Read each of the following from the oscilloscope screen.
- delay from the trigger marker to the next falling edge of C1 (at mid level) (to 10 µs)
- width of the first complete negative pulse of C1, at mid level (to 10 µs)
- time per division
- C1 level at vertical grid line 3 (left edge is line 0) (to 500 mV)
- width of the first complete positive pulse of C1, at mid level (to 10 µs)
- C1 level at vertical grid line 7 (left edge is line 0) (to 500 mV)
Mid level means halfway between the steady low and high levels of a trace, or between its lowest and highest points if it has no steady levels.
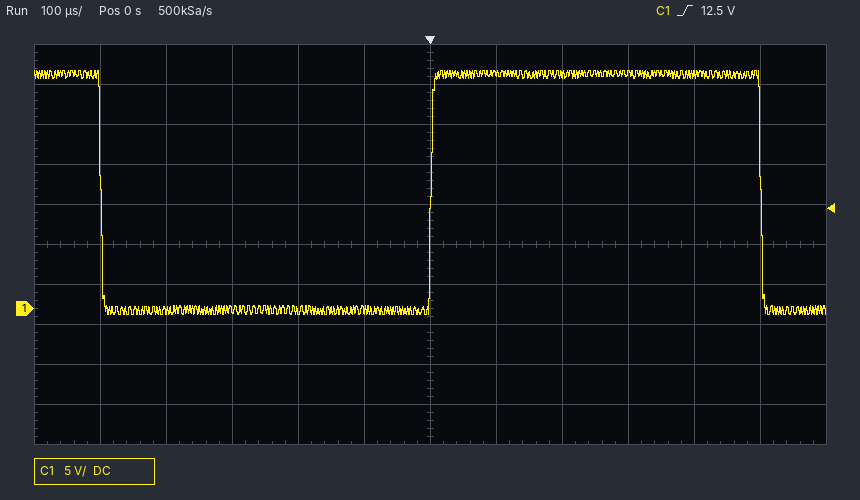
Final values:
500 µs
500 µs
100 µs
0.0 V
500 µs
29.5 V
